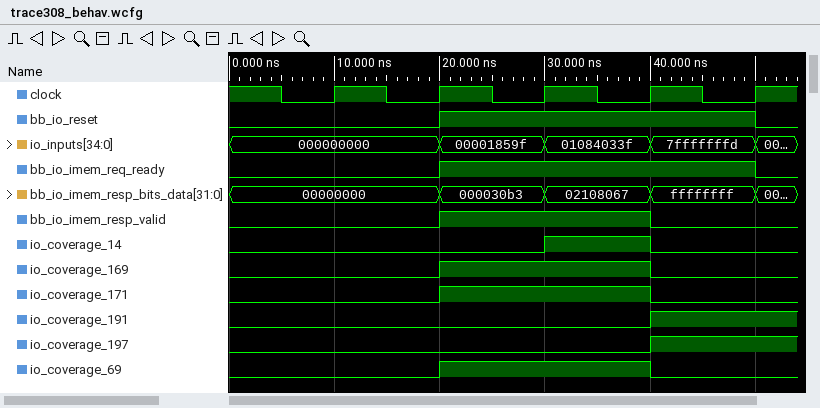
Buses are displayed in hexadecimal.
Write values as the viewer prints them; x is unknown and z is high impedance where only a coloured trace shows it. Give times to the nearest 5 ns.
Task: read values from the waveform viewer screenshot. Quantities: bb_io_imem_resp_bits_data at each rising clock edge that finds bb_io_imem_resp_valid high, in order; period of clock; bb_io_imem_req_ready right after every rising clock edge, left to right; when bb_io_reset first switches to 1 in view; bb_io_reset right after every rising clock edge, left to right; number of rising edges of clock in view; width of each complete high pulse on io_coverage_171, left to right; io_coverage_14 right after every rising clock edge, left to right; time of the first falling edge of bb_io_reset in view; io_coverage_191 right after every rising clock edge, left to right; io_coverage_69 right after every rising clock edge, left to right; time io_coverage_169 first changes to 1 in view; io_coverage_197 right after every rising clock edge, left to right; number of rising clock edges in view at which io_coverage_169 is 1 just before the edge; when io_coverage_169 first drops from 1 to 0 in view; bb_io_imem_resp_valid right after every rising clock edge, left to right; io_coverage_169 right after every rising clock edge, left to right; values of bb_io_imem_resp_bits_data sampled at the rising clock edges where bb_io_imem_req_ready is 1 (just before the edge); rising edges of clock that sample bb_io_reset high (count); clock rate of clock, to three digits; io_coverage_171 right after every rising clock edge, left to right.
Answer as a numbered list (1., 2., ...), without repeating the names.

1. 000030b3, 02108067
2. 10 ns
3. 0 1 1 1 0
4. 20 ns
5. 0 1 1 1 0
6. 5
7. 20 ns
8. 0 0 1 0 0
9. 50 ns
10. 0 0 0 1 1
11. 0 1 1 0 0
12. 20 ns
13. 0 0 0 1 1
14. 2
15. 40 ns
16. 0 1 1 0 0
17. 0 1 1 0 0
18. 000030b3, 02108067, ffffffff
19. 3
20. 100 MHz
21. 0 1 1 0 0
